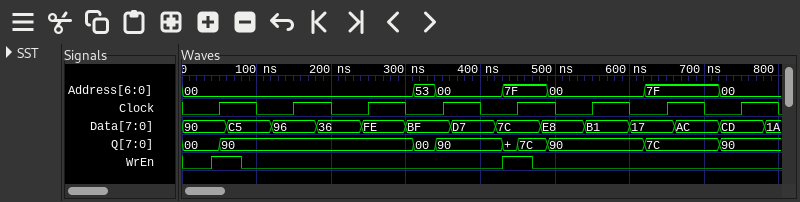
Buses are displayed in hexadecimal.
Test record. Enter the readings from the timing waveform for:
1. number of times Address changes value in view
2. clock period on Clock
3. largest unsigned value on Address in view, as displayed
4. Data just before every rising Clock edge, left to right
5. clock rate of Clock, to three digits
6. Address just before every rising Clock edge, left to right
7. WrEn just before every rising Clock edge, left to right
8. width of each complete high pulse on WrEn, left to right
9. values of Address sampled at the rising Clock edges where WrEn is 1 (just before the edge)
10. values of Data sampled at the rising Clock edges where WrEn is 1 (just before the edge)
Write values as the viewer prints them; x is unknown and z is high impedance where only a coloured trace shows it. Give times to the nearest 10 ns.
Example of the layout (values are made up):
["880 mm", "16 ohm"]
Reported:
["6", "100 ns", "7F", "90, 96, FE, BF, 7C, B1, 17, CD", "10.0 MHz", "00, 00, 00, 00, 7F, 00, 7F, 00", "1 0 0 0 1 0 0 0", "40 ns, 40 ns", "00, 7F", "90, 7C"]
